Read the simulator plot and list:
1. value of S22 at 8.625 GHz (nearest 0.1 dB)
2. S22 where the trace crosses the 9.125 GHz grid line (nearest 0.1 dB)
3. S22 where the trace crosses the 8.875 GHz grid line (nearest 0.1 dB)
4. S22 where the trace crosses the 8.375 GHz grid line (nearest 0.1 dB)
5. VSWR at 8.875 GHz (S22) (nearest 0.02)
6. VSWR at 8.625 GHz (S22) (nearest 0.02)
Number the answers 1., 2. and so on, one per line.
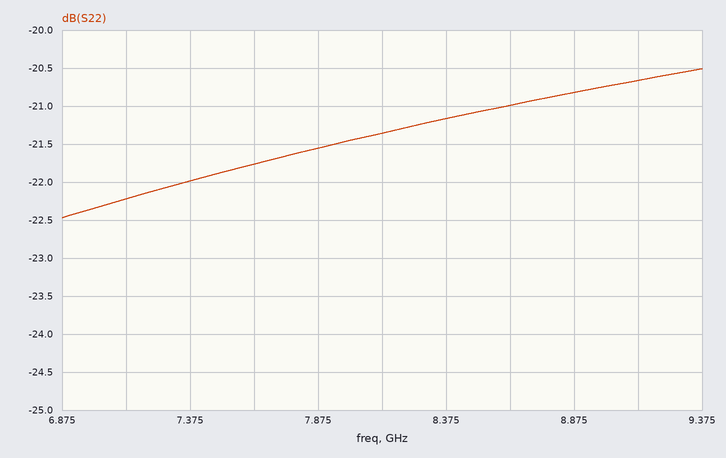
1. -21.0 dB
2. -20.7 dB
3. -20.8 dB
4. -21.2 dB
5. 1.20
6. 1.20
